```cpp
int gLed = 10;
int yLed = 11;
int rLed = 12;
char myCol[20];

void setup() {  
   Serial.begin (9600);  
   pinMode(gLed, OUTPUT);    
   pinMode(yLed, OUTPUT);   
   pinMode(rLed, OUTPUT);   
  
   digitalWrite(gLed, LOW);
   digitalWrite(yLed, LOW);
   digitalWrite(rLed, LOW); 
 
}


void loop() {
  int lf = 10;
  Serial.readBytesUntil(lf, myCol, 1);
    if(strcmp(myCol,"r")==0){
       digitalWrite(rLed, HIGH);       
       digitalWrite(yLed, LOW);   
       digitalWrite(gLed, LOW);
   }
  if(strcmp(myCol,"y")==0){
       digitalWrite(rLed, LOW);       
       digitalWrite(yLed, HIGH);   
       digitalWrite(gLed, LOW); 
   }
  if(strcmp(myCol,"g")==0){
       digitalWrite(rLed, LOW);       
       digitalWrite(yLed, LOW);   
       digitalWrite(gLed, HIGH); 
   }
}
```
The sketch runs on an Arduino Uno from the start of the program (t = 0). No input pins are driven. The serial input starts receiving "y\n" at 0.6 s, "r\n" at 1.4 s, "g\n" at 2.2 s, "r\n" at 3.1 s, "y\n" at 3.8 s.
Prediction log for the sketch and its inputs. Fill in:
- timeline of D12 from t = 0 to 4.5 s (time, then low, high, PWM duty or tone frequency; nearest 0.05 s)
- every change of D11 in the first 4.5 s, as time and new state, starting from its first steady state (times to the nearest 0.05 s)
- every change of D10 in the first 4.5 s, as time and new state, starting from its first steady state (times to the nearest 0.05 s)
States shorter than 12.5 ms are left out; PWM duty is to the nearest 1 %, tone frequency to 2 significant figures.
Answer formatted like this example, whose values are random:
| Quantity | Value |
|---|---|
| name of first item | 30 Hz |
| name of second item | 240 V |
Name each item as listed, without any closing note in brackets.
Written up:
| Quantity | Value |
|---|---|
| timeline of D12 from t = 0 to 4.5 s | 0 s low; 1.4 s high; 2.2 s low; 3.1 s high; 3.8 s low |
| every change of D11 in the first 4.5 s, as time and new state, starting from its first steady state | 0 s low; 0.6 s high; 1.4 s low; 3.8 s high |
| every change of D10 in the first 4.5 s, as time and new state, starting from its first steady state | 0 s low; 2.2 s high; 3.1 s low |
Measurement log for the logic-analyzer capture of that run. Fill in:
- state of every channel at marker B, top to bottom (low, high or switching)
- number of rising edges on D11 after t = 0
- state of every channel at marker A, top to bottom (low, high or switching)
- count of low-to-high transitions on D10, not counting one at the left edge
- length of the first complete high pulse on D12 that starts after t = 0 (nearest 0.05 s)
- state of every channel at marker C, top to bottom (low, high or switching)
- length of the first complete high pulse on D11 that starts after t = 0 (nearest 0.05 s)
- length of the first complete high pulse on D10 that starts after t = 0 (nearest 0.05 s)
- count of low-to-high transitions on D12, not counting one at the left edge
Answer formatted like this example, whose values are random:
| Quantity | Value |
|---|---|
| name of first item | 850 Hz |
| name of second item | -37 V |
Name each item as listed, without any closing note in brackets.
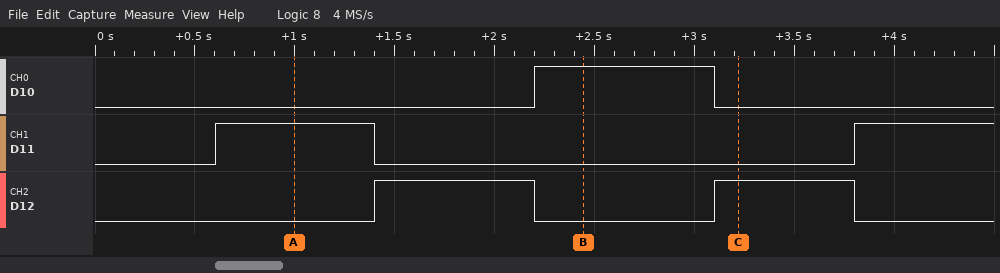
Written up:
| Quantity | Value |
|---|---|
| state of every channel at marker B, top to bottom | D10 high, D11 low, D12 low |
| number of rising edges on D11 after t = 0 | 2 |
| state of every channel at marker A, top to bottom | D10 low, D11 high, D12 low |
| count of low-to-high transitions on D10, not counting one at the left edge | 1 |
| length of the first complete high pulse on D12 that starts after t = 0 | 0.80 s |
| state of every channel at marker C, top to bottom | D10 low, D11 low, D12 high |
| length of the first complete high pulse on D11 that starts after t = 0 | 0.80 s |
| length of the first complete high pulse on D10 that starts after t = 0 | 0.90 s |
| count of low-to-high transitions on D12, not counting one at the left edge | 2 |
